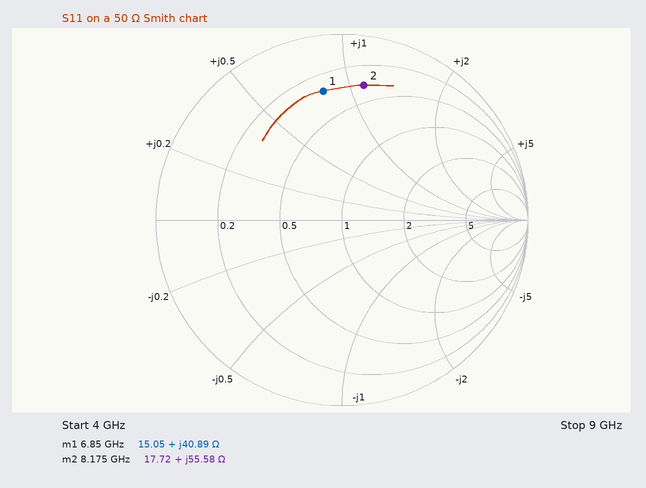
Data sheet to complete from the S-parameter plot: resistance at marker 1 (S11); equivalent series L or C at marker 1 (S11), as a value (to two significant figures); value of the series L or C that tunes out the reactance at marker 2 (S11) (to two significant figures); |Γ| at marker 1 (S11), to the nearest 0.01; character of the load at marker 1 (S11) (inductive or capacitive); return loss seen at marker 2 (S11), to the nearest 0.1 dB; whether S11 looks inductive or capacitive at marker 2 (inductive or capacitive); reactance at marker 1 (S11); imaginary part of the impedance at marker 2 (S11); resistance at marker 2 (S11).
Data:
15.05 Ω
950 pH
350 fF
0.70
inductive
2.7 dB
inductive
+40.89 Ω
+55.58 Ω
17.72 Ω
